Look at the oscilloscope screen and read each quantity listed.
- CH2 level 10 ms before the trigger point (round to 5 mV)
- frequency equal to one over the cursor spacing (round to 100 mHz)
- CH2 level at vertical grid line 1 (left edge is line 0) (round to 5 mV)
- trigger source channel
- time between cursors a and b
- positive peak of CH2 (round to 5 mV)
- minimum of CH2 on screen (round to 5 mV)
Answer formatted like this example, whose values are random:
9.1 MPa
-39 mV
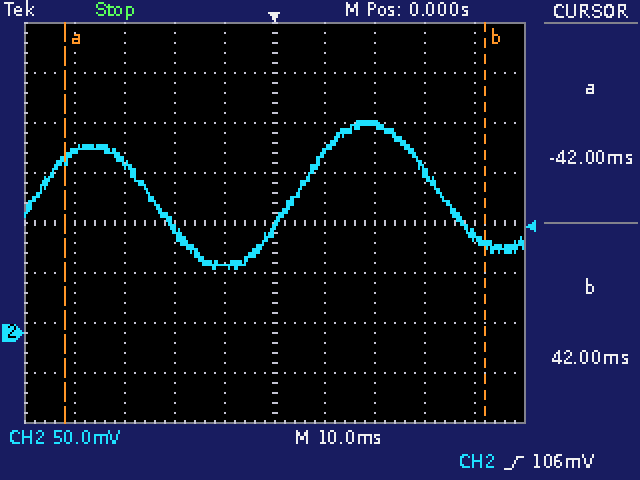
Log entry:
70 mV
11.9 Hz
180 mV
CH2
84 ms
210 mV
65 mV
